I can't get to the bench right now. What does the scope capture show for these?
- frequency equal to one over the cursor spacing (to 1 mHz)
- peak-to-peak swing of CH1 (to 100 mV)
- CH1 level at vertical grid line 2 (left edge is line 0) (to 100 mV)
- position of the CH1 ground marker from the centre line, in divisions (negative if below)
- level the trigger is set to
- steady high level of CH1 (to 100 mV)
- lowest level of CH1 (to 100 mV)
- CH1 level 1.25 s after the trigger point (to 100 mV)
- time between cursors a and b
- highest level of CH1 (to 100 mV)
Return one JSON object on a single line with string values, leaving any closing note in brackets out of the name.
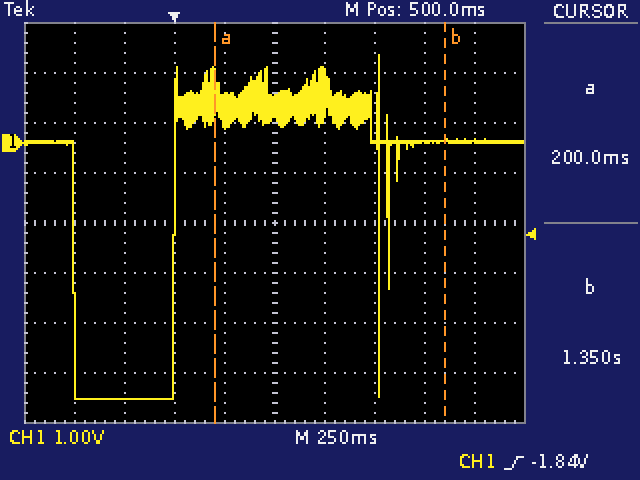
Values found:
{"frequency equal to one over the cursor spacing": "870 mHz", "peak-to-peak swing of CH1": "6.9 V", "CH1 level at vertical grid line 2 (left edge is line 0)": "-5.1 V", "position of the CH1 ground marker from the centre line, in divisions": "+1.6 div", "level the trigger is set to": "-1.84 V", "steady high level of CH1": "0.0 V", "lowest level of CH1": "-5.1 V", "CH1 level 1.25 s after the trigger point": "0.0 V", "time between cursors a and b": "1.150 s", "highest level of CH1": "1.8 V"}
